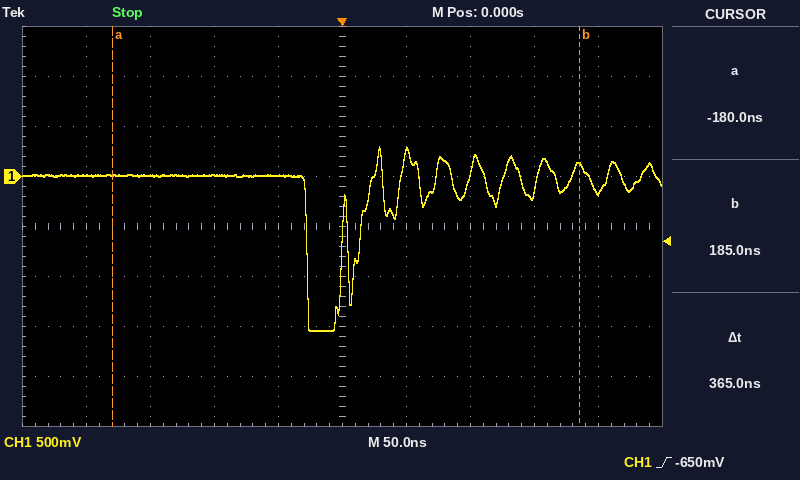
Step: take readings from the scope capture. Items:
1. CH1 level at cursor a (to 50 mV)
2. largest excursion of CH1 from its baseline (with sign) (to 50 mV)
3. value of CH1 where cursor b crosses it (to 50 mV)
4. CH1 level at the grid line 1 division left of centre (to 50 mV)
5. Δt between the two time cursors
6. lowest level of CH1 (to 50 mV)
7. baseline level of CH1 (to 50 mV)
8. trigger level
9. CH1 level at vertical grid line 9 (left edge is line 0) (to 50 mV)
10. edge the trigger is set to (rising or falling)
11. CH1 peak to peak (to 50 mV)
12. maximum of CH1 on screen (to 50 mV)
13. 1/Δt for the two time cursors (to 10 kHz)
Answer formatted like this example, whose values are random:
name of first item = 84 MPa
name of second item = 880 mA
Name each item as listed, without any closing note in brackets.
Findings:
CH1 level at cursor a = 0 mV
largest excursion of CH1 from its baseline (with sign) = -1.55 V
value of CH1 where cursor b crosses it = 100 mV
CH1 level at the grid line 1 division left of centre = 0 mV
Δt between the two time cursors = 365 ns
lowest level of CH1 = -1.55 V
baseline level of CH1 = 0 mV
trigger level = -650 mV
CH1 level at vertical grid line 9 (left edge is line 0) = -150 mV
edge the trigger is set to = rising
CH1 peak to peak = 1.85 V
maximum of CH1 on screen = 300 mV
1/Δt for the two time cursors = 2.74 MHz
